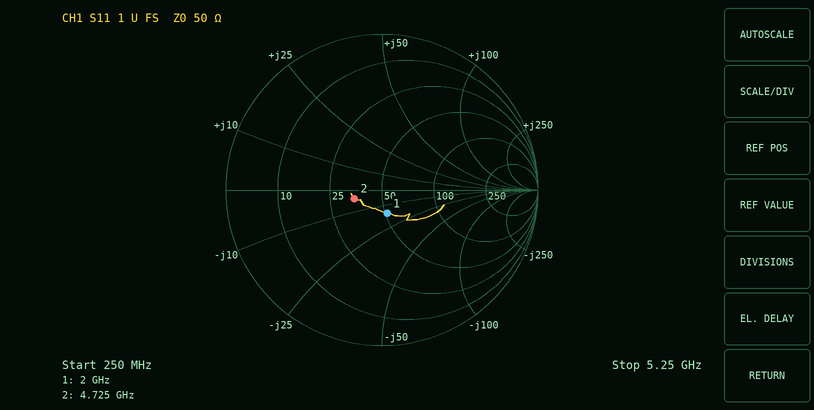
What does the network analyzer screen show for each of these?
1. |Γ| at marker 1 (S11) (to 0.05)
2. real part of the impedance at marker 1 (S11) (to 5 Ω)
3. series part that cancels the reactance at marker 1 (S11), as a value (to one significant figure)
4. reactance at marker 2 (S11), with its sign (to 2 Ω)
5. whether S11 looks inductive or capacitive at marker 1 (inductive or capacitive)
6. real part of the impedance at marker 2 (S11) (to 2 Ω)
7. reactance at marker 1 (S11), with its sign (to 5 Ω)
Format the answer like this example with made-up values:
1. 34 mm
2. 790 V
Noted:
1. 0.15
2. 50 Ω
3. 1 nH
4. -4 Ω
5. capacitive
6. 34 Ω
7. -15 Ω
